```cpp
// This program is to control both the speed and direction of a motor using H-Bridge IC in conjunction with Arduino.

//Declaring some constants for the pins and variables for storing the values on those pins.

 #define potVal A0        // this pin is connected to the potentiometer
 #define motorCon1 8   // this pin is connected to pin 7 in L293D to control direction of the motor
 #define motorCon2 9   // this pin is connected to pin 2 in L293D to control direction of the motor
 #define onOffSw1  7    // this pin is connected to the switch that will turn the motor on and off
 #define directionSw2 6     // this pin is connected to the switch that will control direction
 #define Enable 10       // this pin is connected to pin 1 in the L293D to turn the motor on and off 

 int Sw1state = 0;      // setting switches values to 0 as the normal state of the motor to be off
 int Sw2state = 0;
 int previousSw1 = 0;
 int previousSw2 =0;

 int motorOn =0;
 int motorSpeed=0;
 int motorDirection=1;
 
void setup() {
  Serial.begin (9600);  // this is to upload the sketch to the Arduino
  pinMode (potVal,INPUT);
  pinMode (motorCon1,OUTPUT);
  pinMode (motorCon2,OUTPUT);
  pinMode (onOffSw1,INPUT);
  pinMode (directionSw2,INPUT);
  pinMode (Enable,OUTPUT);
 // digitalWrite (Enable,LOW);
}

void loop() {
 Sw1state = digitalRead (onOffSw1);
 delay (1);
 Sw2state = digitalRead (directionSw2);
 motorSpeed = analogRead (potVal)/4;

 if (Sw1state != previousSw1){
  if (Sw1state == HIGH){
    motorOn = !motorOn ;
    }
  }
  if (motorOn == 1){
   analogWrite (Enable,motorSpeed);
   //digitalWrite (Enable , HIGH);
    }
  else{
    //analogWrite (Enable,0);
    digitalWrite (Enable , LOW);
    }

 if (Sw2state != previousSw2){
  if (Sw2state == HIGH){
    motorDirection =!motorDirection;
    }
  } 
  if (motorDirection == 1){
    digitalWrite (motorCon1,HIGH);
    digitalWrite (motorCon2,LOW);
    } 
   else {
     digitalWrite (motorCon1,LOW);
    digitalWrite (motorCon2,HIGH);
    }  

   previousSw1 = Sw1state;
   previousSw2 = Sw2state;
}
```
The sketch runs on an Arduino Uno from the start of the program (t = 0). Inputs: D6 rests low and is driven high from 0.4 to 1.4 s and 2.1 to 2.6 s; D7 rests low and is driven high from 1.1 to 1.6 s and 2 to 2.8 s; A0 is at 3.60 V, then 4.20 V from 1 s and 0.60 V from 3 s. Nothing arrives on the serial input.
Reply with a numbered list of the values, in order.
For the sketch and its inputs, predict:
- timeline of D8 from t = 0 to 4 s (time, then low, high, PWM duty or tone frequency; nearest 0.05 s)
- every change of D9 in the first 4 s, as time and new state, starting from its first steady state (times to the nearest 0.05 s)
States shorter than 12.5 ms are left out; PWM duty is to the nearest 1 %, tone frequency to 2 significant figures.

1. 0 s high; 0.4 s low; 2.1 s high
2. 0 s low; 0.4 s high; 2.1 s low
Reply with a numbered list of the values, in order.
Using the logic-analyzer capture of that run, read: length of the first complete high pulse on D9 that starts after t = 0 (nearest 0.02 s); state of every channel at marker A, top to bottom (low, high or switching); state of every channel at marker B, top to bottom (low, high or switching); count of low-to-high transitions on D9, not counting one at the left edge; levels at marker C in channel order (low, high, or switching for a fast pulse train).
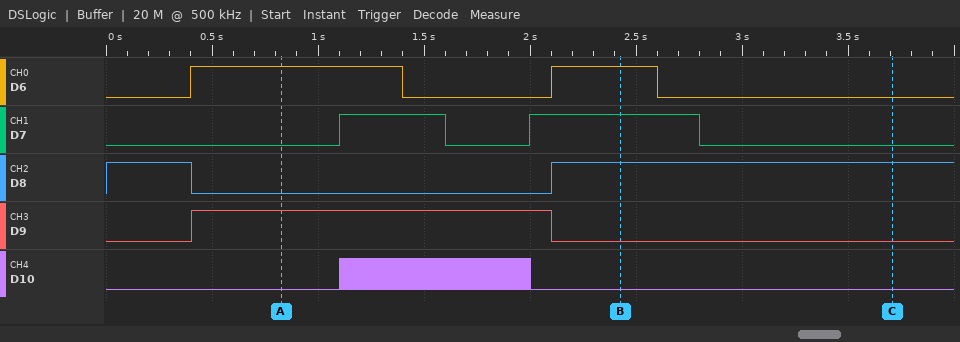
1. 1.70 s
2. D6 high, D7 low, D8 low, D9 high, D10 low
3. D6 high, D7 high, D8 high, D9 low, D10 low
4. 1
5. D6 low, D7 low, D8 high, D9 low, D10 low
